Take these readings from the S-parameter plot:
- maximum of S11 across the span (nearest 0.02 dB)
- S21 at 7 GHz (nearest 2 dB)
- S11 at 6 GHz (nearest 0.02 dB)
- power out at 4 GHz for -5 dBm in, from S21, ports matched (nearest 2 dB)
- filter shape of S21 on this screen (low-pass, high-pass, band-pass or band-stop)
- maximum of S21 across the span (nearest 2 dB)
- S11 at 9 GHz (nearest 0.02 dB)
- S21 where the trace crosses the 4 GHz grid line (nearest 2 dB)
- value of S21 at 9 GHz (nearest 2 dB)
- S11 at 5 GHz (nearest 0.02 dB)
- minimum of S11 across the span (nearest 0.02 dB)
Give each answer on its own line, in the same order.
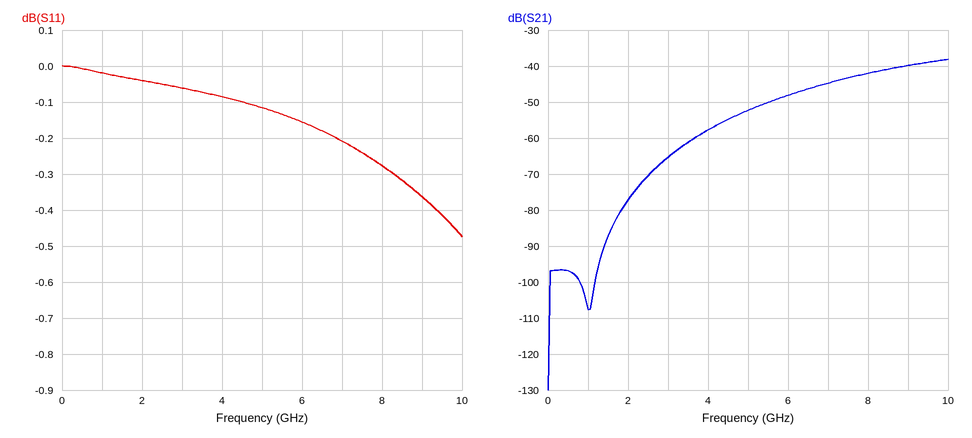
0.00 dB
-44 dB
-0.16 dB
-62 dBm
high-pass
-38 dB
-0.36 dB
-58 dB
-40 dB
-0.12 dB
-0.48 dB
